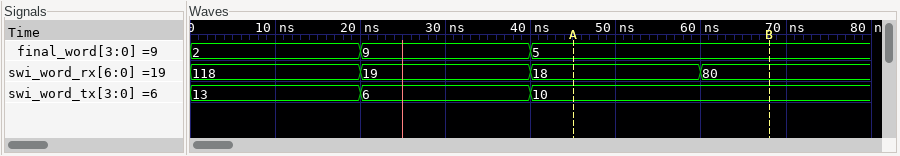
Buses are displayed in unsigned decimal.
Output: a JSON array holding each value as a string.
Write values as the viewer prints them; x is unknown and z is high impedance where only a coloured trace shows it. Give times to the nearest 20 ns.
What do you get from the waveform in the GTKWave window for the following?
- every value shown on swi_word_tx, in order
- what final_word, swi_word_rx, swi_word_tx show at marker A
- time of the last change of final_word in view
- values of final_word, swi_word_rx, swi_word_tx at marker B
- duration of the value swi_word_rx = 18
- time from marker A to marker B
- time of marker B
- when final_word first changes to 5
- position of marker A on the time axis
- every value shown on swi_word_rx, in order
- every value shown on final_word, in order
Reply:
["13, 6, 10", "final_word=5, swi_word_rx=18, swi_word_tx=10", "40 ns", "final_word=5, swi_word_rx=80, swi_word_tx=10", "20 ns", "20 ns", "60 ns", "40 ns", "40 ns", "118, 19, 18, 80", "2, 9, 5"]
